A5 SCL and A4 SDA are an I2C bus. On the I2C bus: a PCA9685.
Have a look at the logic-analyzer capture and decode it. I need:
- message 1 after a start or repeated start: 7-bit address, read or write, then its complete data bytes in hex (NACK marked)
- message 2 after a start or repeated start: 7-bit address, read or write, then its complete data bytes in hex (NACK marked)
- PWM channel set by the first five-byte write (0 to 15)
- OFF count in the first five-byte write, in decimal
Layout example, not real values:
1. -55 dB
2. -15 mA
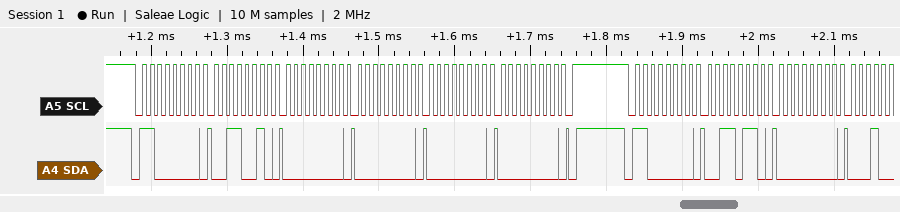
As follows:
1. 0x60 write: 32 00 00 00 00
2. 0x60 write: 36 00
3. 11
4. 0
